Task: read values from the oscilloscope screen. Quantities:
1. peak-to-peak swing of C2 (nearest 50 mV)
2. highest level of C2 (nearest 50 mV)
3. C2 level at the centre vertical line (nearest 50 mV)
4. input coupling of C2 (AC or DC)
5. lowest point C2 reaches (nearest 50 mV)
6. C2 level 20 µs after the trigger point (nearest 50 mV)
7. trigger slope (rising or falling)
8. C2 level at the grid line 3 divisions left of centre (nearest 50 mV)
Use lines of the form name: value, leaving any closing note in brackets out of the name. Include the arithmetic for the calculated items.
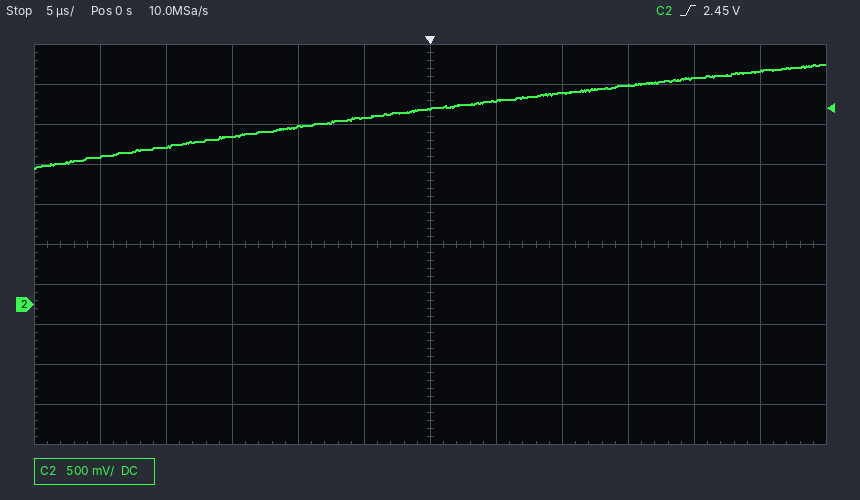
peak-to-peak swing of C2: 3.00 V − (1.70 V) = 1.30 V
highest level of C2: 3.00 V
C2 level at the centre vertical line: 2.45 V
input coupling of C2: DC
lowest point C2 reaches: 1.70 V
C2 level 20 µs after the trigger point: 2.85 V
trigger slope: rising
C2 level at the grid line 3 divisions left of centre: 2.10 V
